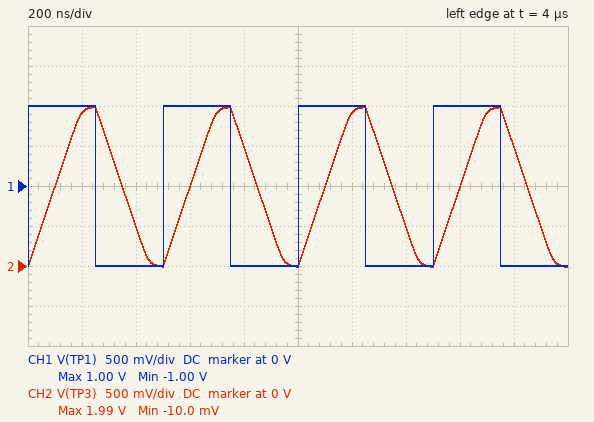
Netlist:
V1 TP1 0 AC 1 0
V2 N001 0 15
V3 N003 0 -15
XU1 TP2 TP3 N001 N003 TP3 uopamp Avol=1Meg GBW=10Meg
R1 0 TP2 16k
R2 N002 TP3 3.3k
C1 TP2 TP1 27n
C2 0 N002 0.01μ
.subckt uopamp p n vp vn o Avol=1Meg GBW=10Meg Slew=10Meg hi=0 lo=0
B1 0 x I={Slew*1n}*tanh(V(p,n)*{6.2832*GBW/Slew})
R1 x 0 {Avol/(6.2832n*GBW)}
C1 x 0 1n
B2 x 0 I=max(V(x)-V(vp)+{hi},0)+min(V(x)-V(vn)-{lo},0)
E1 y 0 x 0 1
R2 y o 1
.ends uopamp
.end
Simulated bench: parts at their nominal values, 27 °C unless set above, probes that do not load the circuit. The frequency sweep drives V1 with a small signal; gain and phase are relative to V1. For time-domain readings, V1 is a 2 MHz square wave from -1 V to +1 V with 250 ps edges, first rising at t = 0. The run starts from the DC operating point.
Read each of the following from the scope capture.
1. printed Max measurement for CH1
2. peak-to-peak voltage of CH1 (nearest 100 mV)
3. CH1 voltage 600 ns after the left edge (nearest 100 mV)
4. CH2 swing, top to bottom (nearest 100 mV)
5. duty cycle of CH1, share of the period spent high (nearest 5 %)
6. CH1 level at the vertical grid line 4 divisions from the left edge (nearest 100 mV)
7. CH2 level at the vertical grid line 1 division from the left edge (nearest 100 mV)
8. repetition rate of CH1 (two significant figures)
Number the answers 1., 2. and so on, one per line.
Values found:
1. 1.00 V
2. 2.0 V
3. 1.0 V
4. 2.0 V
5. 50 %
6. -1.0 V
7. 1.9 V
8. 2.0 MHz
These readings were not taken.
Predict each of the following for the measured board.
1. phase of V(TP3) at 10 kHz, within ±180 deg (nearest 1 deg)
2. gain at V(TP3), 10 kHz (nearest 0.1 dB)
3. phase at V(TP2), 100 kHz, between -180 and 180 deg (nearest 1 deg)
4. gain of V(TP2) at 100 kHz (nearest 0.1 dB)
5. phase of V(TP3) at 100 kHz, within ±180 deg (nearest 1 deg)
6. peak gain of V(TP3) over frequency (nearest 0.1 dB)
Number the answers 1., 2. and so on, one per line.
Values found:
1. 2 deg
2. 0 dB
3. 0 deg
4. 0 dB
5. 0 deg
6. 0 dB
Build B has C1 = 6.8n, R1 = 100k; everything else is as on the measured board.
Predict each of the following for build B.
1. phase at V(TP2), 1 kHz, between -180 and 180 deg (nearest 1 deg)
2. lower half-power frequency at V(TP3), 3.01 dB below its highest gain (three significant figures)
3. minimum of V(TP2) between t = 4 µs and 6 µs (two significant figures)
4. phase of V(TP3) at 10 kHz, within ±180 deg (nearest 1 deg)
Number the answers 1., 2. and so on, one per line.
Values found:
1. 13 deg
2. 234 Hz
3. -8.8 mV
4. 1 deg
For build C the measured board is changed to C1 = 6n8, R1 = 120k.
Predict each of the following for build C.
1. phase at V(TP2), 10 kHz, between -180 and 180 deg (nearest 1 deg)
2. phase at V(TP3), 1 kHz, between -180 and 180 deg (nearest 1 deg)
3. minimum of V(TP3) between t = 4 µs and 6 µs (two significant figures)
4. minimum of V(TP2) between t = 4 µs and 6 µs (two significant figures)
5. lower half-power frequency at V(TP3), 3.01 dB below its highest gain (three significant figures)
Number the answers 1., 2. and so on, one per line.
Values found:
1. 1 deg
2. 11 deg
3. -4.0 mV
4. -7.3 mV
5. 195 Hz
